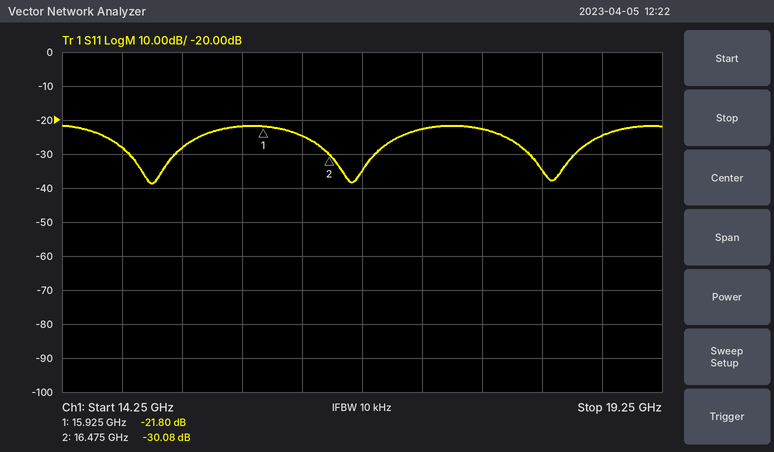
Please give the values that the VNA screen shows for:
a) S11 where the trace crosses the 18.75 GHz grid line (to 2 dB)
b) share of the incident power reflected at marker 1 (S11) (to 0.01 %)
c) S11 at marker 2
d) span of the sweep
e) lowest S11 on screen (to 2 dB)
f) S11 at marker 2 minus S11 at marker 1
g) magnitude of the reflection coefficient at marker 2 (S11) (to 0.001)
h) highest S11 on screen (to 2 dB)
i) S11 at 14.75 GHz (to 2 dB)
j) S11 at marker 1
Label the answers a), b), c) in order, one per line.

a) -24 dB
b) 0.66 %
c) -30.08 dB
d) 5 GHz
e) -38 dB
f) -8.28 dB
g) 0.031
h) -22 dB
i) -28 dB
j) -21.80 dB
